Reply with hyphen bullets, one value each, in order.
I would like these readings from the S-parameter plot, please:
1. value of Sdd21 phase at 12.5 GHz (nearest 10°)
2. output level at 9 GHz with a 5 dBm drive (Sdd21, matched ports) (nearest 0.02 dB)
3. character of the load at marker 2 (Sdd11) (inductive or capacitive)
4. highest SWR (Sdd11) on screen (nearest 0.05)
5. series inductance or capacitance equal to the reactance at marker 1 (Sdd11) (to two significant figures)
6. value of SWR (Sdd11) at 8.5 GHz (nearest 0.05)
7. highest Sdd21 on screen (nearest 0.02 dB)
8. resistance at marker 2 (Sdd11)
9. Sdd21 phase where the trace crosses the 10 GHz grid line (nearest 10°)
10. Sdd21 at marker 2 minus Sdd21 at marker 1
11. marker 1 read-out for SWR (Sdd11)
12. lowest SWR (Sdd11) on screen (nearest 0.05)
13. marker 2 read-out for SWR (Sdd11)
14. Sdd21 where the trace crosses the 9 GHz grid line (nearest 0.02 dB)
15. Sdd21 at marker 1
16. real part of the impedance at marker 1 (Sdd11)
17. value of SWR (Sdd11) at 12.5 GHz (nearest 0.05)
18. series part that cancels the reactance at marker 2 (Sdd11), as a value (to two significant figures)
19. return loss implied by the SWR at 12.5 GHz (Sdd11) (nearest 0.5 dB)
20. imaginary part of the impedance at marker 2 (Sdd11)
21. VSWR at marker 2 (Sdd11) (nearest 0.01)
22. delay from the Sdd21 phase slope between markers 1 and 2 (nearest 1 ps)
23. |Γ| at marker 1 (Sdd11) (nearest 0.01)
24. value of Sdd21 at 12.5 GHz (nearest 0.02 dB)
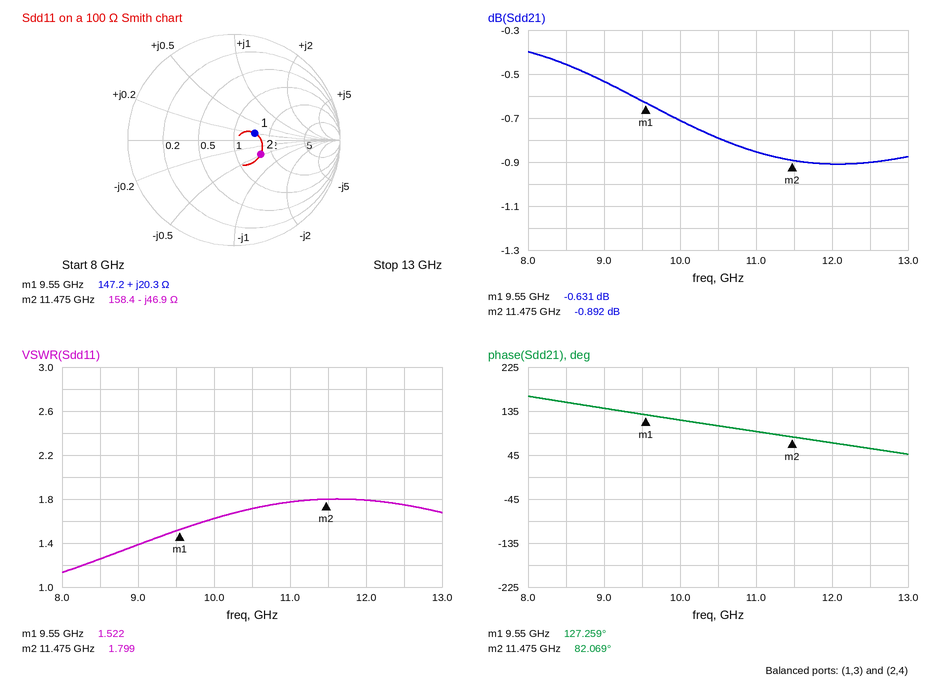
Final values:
- 60°
- 4.46 dBm
- capacitive
- 1.80
- 340 pH
- 1.25
- -0.40 dB
- 158.4 Ω
- 120°
- -0.261 dB
- 1.522
- 1.15
- 1.799
- -0.54 dB
- -0.631 dB
- 147.2 Ω
- 1.75
- 650 pH
- 11.5 dB
- -46.9 Ω
- 1.80
- 65 ps
- 0.21
- -0.90 dB
